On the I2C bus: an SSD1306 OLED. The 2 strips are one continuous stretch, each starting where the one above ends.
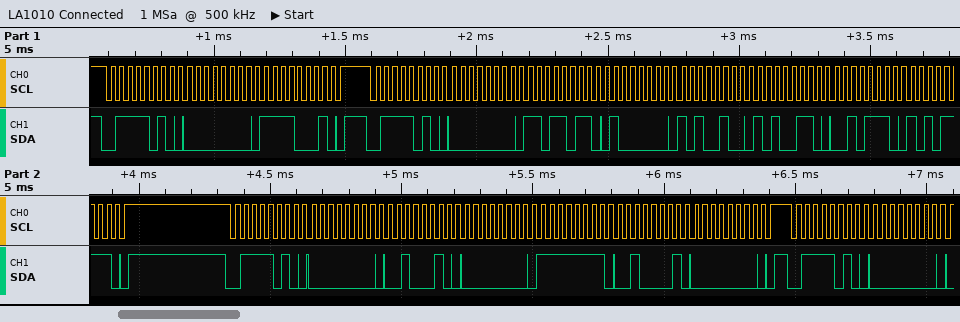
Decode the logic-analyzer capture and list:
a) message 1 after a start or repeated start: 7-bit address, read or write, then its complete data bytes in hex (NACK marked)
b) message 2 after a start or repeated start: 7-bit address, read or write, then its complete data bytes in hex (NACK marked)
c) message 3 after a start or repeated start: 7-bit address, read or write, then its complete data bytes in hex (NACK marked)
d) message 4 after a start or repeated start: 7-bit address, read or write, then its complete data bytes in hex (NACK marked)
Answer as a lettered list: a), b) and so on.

a) 0x3D write: 00 F1
b) 0x3D write: 00 DB 40 A4 A6 2E AF
c) 0x3D write: 00 22 00 FF 21 00
d) 0x3D write: 00
